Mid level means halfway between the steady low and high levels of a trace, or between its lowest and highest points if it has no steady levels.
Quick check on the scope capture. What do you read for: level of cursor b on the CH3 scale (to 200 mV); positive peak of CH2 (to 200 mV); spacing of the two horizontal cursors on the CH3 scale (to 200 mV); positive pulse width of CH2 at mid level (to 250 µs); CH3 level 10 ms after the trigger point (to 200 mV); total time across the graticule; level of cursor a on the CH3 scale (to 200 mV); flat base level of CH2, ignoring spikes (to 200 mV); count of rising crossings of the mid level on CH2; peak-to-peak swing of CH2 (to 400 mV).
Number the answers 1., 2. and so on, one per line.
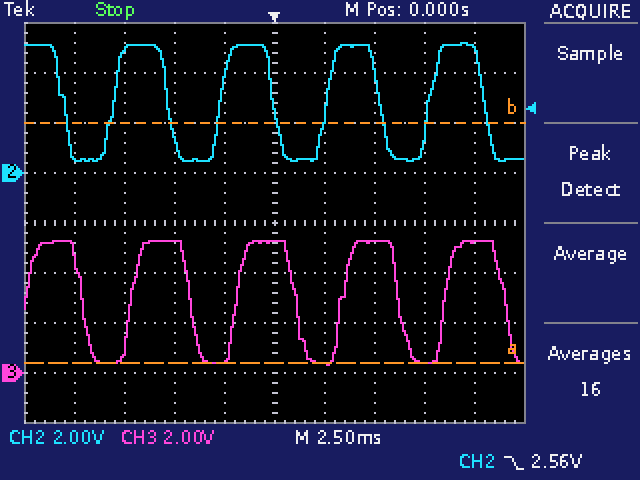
1. 10.0 V
2. 5.2 V
3. 9.6 V
4. 2.75 ms
5. 5.2 V
6. 25 ms
7. 400 mV
8. 600 mV
9. 4
10. 4.8 V
